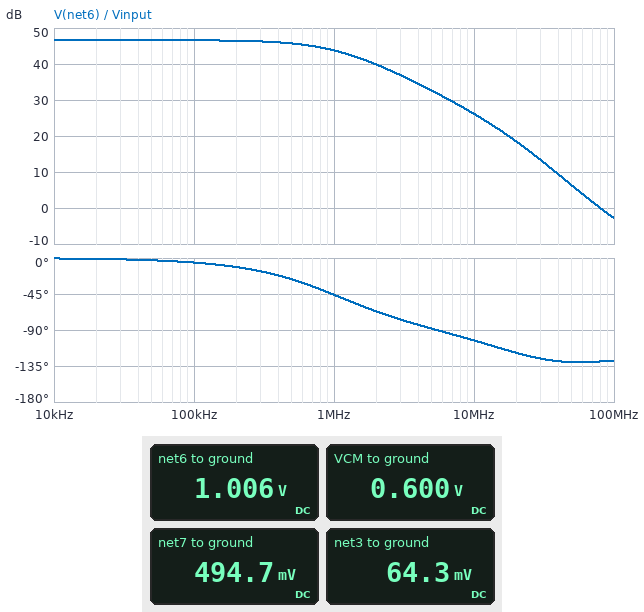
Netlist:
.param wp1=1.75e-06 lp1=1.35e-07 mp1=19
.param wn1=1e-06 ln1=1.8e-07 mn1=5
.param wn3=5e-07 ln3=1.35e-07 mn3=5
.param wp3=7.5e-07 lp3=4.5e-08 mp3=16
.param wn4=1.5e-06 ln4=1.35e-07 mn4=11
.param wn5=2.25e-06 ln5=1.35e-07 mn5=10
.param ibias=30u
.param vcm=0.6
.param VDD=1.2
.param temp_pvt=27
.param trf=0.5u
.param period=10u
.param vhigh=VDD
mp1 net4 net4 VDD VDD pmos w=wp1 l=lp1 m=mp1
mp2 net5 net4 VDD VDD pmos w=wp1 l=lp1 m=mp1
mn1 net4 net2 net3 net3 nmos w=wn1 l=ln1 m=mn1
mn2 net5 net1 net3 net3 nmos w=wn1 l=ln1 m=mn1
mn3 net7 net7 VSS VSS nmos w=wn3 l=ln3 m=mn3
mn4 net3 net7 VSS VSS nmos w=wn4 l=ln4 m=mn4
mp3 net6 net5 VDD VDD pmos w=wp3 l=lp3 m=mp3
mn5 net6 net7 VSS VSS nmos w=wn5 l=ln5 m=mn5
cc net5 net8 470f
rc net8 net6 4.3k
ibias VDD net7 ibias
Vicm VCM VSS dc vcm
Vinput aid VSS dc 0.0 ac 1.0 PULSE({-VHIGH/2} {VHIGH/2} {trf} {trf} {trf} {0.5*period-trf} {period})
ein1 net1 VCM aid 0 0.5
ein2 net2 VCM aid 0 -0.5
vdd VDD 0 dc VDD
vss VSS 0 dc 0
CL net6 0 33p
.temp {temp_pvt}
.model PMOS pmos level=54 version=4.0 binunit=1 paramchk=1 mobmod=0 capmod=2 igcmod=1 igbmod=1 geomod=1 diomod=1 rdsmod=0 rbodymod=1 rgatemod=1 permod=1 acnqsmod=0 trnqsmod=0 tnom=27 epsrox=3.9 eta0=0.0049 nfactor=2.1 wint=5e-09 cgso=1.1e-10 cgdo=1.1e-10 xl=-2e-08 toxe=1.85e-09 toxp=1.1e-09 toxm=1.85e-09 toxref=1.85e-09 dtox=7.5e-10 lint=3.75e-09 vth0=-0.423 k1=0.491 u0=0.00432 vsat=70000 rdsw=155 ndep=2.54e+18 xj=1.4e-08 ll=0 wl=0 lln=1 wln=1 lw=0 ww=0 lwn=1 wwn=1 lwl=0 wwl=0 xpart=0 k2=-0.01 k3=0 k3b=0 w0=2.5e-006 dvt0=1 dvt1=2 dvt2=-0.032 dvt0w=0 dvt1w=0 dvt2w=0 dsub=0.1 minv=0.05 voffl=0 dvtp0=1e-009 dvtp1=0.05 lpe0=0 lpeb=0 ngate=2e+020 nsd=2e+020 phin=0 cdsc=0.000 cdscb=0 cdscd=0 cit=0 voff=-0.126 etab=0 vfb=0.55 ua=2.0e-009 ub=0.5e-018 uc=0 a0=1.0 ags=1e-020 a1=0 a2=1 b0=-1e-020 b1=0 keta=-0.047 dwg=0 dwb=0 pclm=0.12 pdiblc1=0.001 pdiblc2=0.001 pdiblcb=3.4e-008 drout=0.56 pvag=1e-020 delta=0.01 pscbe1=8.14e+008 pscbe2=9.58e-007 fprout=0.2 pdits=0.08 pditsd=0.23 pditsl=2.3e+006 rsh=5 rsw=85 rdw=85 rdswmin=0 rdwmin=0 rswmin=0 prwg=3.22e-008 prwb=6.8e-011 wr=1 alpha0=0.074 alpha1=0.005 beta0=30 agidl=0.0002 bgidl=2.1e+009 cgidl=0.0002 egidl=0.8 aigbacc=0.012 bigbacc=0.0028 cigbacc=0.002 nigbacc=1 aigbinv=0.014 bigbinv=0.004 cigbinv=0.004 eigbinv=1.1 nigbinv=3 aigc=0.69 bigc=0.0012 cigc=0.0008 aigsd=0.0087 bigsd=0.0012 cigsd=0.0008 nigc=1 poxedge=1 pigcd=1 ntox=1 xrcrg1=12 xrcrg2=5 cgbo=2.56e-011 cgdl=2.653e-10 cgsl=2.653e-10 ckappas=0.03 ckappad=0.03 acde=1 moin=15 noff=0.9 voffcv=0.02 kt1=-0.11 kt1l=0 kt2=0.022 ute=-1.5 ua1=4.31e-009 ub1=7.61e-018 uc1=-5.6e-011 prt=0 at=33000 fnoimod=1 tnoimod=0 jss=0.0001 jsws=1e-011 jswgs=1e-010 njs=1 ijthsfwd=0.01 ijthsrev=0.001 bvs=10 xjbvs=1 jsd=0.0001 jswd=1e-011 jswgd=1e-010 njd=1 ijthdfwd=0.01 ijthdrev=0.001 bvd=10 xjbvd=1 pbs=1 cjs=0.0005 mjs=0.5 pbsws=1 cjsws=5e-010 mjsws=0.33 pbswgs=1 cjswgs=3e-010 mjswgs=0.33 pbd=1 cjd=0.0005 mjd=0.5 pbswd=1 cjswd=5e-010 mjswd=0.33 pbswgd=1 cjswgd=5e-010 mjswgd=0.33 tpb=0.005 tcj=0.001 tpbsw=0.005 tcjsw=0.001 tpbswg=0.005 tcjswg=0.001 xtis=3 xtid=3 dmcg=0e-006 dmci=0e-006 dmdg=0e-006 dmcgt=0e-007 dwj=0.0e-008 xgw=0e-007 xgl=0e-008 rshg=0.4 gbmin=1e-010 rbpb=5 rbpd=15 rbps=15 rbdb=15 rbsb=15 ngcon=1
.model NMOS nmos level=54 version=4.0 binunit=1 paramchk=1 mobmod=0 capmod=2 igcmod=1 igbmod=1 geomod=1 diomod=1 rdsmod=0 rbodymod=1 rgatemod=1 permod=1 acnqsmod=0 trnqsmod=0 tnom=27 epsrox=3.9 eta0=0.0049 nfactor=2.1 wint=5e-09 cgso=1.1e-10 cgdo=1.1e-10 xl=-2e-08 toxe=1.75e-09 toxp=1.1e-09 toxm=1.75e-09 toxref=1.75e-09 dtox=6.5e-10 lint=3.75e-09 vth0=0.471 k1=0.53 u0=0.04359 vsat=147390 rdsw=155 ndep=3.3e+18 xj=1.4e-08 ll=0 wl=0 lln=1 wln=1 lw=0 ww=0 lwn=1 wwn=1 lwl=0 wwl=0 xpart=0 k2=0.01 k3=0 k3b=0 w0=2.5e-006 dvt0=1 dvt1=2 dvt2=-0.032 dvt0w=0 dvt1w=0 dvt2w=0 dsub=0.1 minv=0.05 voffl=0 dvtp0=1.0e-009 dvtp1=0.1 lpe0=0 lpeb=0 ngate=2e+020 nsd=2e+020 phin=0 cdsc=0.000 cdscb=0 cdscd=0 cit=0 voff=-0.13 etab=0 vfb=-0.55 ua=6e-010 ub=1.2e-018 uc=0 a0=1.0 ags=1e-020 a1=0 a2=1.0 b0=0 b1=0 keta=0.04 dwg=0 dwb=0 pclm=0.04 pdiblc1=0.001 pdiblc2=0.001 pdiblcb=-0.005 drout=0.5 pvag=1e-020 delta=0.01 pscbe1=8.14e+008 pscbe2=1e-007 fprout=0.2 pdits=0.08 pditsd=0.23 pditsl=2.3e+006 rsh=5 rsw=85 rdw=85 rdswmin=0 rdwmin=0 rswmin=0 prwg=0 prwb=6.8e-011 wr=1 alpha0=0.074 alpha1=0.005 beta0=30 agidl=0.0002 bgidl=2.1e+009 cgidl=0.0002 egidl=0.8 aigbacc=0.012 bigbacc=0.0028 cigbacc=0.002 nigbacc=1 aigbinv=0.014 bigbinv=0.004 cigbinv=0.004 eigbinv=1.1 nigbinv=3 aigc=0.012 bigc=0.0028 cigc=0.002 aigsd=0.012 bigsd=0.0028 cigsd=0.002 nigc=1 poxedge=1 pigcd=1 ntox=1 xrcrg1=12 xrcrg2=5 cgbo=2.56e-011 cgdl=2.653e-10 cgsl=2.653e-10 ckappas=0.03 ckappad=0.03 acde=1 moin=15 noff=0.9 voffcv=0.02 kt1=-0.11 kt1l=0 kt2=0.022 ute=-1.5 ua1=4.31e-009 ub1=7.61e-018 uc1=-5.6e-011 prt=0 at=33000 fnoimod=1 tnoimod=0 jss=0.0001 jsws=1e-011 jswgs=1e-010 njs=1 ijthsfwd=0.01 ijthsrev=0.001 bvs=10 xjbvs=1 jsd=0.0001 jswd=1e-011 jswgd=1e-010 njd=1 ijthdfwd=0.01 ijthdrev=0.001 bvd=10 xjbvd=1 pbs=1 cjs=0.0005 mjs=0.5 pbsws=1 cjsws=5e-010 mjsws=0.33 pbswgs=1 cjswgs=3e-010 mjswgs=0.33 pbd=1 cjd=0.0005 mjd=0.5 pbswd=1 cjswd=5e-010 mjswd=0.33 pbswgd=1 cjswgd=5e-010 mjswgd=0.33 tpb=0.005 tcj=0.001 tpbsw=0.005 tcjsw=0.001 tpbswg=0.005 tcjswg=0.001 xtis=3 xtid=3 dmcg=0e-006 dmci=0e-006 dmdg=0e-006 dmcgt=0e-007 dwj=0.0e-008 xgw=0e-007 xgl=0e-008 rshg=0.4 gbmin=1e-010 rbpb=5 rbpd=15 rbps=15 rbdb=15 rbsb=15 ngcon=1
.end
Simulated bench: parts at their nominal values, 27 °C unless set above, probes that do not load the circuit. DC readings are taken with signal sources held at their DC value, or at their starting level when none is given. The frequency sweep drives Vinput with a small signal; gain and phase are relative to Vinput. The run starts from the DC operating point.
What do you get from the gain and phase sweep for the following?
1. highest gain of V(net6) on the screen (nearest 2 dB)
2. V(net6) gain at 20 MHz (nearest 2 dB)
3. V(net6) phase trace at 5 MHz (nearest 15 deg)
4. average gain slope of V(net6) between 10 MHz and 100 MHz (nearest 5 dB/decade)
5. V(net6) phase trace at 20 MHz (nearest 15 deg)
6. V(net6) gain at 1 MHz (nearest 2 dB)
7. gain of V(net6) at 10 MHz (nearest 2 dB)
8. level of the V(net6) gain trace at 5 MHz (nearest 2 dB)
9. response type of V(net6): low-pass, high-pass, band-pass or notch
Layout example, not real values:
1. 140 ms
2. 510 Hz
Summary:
1. 46 dB
2. 18 dB
3. -90 deg
4. -30 dB/decade
5. -120 deg
6. 44 dB
7. 26 dB
8. 32 dB
9. low-pass
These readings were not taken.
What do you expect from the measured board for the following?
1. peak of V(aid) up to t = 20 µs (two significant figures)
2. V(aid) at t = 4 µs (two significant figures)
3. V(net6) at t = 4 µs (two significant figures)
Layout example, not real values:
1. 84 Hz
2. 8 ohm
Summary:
1. 600 mV
2. 600 mV
3. 1.2 V
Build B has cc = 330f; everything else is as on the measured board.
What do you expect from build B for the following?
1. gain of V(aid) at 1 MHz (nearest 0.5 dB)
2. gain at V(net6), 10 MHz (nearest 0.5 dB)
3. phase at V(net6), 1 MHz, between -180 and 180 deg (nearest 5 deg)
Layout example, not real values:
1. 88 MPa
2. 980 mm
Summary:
1. 0 dB
2. 28.5 dB
3. -40 deg
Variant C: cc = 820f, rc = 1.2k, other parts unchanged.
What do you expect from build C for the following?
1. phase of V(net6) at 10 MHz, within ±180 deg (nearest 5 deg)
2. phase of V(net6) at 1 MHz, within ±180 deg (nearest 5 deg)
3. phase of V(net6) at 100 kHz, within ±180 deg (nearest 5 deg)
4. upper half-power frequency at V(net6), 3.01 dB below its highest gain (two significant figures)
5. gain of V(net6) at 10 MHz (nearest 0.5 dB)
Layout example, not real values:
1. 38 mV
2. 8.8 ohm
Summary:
1. -110 deg
2. -60 deg
3. -10 deg
4. 660 kHz
5. 22.0 dB
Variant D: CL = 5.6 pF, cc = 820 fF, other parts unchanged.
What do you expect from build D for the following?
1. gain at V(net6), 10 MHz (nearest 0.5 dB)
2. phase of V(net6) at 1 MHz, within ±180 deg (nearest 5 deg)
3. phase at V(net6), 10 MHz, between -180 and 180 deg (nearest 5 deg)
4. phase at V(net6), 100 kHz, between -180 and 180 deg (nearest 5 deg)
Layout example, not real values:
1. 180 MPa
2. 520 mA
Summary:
1. 24.0 dB
2. -55 deg
3. -80 deg
4. -10 deg
